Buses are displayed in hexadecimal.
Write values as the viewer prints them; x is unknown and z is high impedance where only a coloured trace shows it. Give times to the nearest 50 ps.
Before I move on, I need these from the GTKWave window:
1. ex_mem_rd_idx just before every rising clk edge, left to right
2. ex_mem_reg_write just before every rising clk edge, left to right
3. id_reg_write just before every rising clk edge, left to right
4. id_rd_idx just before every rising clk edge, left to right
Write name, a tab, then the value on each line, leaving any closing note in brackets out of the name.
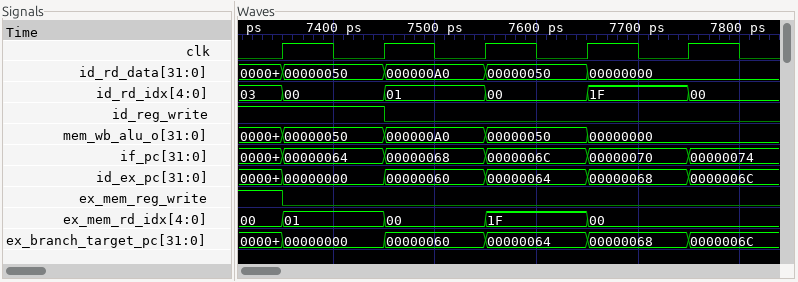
ex_mem_rd_idx just before every rising clk edge, left to right	00, 01, 00, 1F, 00
ex_mem_reg_write just before every rising clk edge, left to right	1 0 0 0 0
id_reg_write just before every rising clk edge, left to right	1 1 0 0 0
id_rd_idx just before every rising clk edge, left to right	03, 00, 01, 00, 1F
